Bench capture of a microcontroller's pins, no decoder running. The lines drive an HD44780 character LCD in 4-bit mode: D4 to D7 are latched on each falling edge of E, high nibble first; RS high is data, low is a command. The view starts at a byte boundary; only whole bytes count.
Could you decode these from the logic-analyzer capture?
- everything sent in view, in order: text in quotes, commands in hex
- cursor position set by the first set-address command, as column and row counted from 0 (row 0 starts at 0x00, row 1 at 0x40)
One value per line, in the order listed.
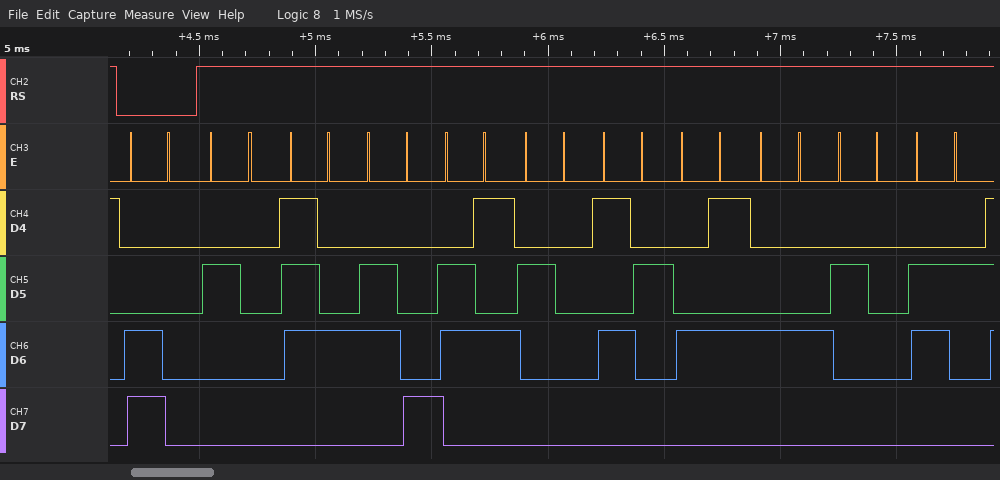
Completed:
0xC0 " the RED b"
column 0, row 1
